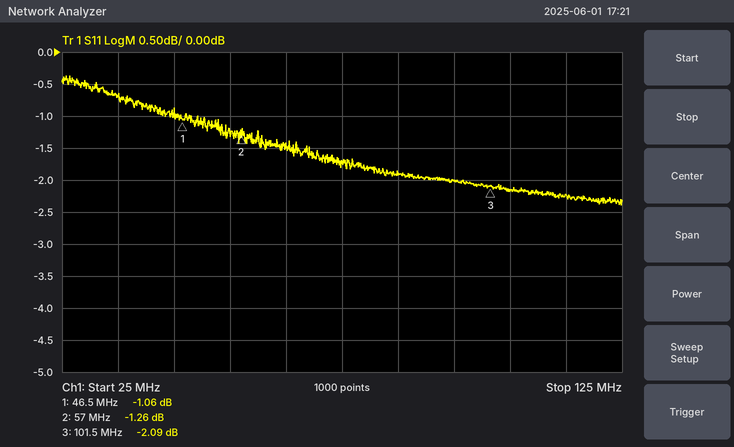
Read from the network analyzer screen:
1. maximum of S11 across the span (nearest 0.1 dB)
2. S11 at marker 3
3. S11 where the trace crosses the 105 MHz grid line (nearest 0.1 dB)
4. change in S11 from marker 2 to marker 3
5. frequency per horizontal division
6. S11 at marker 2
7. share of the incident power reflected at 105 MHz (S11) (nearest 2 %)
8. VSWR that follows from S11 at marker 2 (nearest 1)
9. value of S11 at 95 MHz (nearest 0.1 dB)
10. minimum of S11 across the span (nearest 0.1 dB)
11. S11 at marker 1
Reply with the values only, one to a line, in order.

-0.4 dB
-2.09 dB
-2.2 dB
-0.83 dB
10 MHz
-1.26 dB
60 %
14
-2.0 dB
-2.4 dB
-1.06 dB
